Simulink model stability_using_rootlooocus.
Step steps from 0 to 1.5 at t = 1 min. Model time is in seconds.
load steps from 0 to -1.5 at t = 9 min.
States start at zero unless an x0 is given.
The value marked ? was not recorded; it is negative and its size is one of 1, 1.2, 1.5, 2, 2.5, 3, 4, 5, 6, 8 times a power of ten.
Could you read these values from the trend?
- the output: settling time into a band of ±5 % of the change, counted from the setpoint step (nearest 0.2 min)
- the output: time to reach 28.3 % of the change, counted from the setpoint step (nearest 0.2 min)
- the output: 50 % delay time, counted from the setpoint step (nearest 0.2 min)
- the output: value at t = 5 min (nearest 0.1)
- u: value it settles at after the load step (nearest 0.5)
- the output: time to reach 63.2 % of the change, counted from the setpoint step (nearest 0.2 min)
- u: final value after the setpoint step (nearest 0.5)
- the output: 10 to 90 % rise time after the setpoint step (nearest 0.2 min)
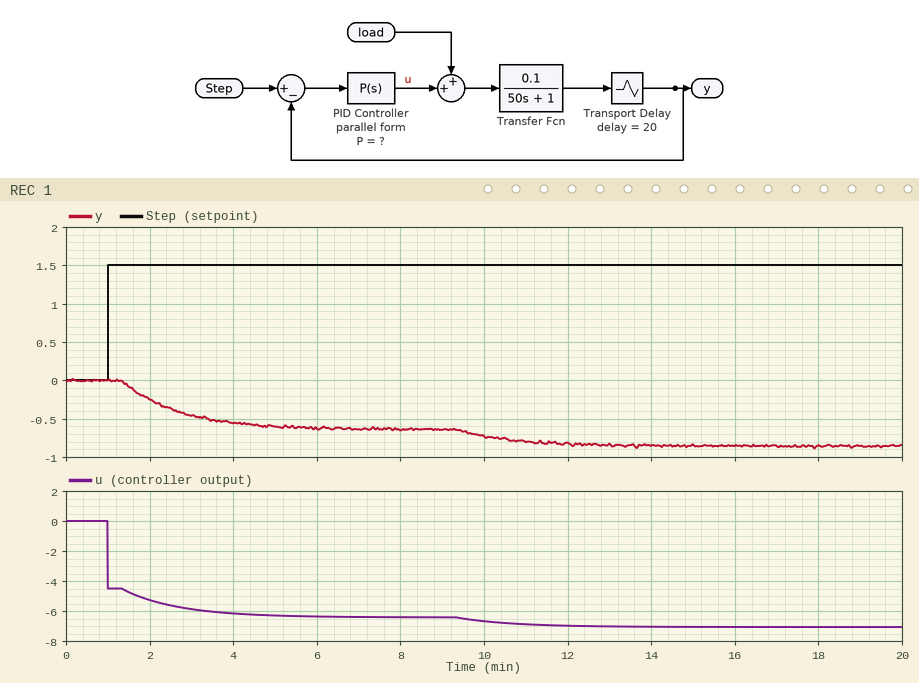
4.4 min
0.8 min
1.2 min
-0.6
-7.0
1.6 min
-6.5
3.0 min
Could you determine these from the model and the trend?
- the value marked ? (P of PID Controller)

-3
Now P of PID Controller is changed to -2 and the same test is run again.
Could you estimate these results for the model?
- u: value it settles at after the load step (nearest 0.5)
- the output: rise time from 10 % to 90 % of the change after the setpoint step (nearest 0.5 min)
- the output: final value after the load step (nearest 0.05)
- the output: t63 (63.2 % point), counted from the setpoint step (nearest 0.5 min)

-4.0
2.5 min
-0.55
1.5 min
